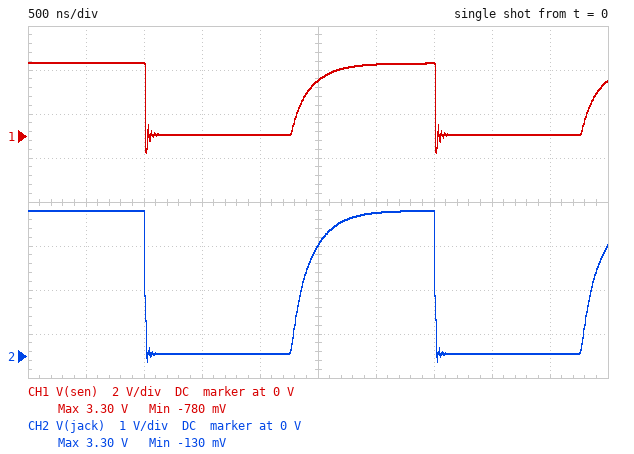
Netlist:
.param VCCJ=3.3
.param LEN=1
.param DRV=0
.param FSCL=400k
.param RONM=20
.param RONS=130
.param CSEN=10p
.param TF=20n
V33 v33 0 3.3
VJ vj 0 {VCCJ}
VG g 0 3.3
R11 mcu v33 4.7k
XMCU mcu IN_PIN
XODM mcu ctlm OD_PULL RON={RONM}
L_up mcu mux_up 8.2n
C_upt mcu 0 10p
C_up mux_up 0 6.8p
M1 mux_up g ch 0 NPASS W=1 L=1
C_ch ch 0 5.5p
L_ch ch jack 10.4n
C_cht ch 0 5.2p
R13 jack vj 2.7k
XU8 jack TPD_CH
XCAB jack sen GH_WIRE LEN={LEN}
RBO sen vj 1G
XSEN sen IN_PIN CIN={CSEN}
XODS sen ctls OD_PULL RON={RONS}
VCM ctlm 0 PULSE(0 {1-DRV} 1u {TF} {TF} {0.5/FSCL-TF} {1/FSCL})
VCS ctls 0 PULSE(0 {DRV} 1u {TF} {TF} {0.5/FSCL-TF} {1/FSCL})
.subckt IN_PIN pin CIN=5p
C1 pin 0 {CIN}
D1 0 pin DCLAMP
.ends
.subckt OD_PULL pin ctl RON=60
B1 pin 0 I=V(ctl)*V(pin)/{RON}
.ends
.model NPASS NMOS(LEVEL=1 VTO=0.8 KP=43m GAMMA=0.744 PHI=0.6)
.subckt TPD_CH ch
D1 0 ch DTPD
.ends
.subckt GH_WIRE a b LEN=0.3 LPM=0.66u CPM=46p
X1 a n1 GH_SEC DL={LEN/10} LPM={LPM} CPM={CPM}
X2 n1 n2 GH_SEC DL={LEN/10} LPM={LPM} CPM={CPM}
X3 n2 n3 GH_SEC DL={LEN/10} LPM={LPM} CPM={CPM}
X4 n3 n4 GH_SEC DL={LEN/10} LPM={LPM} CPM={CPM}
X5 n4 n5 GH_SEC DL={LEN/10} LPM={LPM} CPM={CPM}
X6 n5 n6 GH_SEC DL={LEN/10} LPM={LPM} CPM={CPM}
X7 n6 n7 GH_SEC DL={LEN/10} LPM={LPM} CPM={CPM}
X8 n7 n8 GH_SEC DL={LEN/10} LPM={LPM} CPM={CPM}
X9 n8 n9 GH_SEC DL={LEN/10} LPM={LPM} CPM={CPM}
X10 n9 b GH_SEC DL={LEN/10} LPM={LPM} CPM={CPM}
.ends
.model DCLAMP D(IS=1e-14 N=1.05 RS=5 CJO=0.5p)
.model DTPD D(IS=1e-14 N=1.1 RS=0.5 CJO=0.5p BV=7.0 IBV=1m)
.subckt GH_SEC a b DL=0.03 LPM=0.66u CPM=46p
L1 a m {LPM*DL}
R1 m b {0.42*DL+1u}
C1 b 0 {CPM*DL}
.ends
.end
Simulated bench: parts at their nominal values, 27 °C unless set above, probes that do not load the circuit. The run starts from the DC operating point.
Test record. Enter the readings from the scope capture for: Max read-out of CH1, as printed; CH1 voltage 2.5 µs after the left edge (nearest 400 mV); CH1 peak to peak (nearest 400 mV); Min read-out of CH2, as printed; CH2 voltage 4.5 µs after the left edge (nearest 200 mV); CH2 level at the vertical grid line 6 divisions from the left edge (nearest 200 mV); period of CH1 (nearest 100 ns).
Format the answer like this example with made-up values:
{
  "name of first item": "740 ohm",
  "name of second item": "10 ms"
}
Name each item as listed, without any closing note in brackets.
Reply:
{
  "Max read-out of CH1, as printed": "3.30 V",
  "CH1 voltage 2.5 µs after the left edge": "2.4 V",
  "CH1 peak to peak": "4.0 V",
  "Min read-out of CH2, as printed": "-130 mV",
  "CH2 voltage 4.5 µs after the left edge": "0 V",
  "CH2 level at the vertical grid line 6 divisions from the left edge": "3.2 V",
  "period of CH1": "2.5 µs"
}
